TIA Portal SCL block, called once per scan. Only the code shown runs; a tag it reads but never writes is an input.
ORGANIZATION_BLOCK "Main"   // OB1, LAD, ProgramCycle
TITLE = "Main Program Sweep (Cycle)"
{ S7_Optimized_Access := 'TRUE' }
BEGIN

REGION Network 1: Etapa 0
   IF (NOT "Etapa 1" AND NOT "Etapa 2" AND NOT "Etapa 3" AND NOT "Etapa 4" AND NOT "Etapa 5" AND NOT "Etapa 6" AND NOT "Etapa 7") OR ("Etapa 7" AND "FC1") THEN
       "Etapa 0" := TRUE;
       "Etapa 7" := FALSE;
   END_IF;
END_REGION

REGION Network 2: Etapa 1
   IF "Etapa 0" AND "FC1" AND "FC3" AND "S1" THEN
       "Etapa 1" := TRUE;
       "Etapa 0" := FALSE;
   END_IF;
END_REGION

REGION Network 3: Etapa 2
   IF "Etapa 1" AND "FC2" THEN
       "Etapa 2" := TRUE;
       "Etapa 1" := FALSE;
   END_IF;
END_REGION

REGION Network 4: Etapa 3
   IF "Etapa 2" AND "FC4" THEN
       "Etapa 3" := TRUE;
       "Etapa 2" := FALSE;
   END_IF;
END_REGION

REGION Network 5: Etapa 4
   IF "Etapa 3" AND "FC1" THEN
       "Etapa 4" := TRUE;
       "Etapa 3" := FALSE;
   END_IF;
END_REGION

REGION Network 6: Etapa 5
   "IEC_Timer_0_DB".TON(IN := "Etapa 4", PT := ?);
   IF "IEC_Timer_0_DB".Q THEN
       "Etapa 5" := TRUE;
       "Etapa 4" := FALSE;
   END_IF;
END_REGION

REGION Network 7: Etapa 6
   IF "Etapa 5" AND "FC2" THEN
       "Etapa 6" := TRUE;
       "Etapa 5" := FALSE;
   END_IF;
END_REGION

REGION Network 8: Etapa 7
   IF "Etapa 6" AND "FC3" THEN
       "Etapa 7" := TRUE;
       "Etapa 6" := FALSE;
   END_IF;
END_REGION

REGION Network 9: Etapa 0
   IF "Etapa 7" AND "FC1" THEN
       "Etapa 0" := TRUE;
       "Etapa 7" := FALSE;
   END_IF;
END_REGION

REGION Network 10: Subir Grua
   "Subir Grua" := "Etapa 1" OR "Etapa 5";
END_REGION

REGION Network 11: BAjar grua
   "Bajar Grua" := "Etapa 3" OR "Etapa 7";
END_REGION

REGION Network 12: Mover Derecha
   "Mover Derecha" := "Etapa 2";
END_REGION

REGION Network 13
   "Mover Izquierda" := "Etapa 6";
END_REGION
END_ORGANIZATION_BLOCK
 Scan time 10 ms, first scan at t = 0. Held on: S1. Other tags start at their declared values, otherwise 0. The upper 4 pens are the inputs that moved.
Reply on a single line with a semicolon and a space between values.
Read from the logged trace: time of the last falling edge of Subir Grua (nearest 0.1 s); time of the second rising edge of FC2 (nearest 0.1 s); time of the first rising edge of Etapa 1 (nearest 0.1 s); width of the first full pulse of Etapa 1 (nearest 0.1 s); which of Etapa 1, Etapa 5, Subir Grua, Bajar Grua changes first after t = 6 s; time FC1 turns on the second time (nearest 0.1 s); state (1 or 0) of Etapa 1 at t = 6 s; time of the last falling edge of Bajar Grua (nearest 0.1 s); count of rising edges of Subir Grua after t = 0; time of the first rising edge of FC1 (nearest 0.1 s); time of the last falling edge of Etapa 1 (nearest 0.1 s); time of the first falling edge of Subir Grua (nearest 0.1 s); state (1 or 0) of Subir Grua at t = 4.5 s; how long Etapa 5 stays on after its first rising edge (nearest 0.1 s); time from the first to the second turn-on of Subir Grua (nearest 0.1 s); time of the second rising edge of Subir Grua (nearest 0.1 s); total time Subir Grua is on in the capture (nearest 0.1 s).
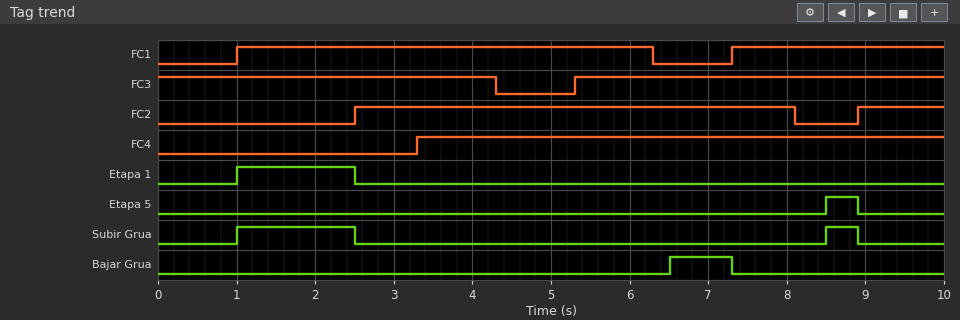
8.9 s; 8.9 s; 1.0 s; 1.5 s; Bajar Grua; 7.3 s; 0; 7.3 s; 2; 1.0 s; 2.5 s; 2.5 s; 0; 0.4 s; 7.5 s; 8.5 s; 1.9 s
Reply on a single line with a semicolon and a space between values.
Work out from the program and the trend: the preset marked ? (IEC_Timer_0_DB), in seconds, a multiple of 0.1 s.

1.2 s
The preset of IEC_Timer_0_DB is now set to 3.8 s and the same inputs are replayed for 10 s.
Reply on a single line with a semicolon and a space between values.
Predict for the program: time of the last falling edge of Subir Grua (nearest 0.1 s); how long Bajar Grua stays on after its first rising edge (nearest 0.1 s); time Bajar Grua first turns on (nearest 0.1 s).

2.5 s; 0.2 s; 7.1 s
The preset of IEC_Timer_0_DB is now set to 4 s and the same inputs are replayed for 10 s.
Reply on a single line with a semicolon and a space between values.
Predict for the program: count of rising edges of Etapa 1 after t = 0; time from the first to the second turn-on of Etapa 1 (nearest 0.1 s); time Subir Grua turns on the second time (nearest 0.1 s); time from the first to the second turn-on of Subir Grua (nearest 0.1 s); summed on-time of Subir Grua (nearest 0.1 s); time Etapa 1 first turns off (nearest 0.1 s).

2; 7.1 s; 8.1 s; 7.1 s; 2.3 s; 2.5 s
